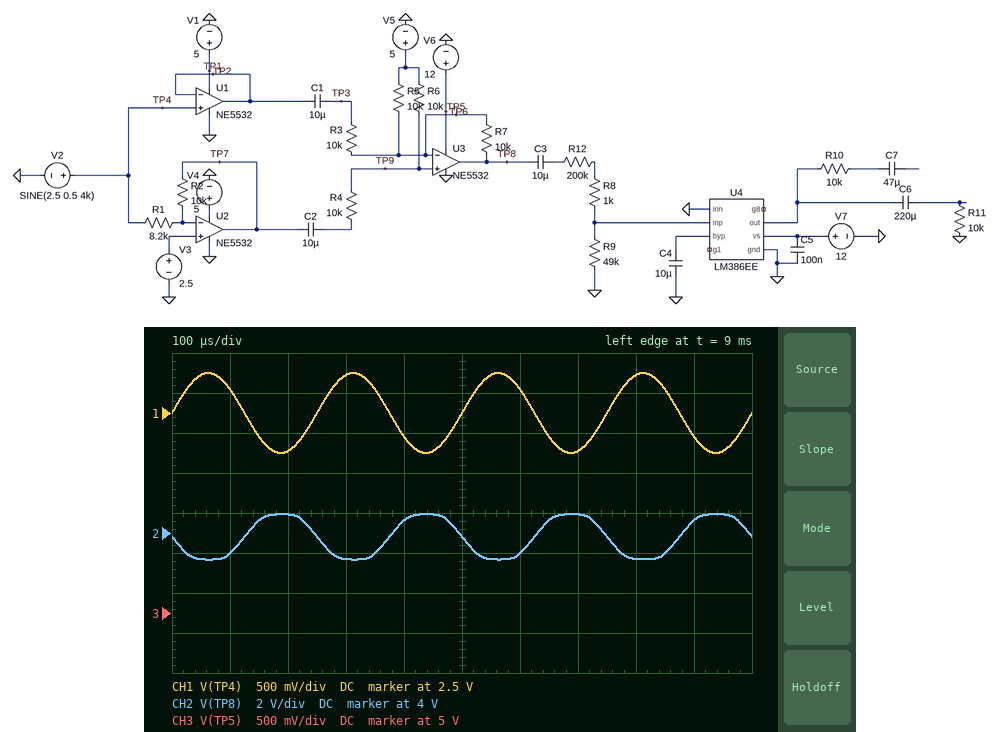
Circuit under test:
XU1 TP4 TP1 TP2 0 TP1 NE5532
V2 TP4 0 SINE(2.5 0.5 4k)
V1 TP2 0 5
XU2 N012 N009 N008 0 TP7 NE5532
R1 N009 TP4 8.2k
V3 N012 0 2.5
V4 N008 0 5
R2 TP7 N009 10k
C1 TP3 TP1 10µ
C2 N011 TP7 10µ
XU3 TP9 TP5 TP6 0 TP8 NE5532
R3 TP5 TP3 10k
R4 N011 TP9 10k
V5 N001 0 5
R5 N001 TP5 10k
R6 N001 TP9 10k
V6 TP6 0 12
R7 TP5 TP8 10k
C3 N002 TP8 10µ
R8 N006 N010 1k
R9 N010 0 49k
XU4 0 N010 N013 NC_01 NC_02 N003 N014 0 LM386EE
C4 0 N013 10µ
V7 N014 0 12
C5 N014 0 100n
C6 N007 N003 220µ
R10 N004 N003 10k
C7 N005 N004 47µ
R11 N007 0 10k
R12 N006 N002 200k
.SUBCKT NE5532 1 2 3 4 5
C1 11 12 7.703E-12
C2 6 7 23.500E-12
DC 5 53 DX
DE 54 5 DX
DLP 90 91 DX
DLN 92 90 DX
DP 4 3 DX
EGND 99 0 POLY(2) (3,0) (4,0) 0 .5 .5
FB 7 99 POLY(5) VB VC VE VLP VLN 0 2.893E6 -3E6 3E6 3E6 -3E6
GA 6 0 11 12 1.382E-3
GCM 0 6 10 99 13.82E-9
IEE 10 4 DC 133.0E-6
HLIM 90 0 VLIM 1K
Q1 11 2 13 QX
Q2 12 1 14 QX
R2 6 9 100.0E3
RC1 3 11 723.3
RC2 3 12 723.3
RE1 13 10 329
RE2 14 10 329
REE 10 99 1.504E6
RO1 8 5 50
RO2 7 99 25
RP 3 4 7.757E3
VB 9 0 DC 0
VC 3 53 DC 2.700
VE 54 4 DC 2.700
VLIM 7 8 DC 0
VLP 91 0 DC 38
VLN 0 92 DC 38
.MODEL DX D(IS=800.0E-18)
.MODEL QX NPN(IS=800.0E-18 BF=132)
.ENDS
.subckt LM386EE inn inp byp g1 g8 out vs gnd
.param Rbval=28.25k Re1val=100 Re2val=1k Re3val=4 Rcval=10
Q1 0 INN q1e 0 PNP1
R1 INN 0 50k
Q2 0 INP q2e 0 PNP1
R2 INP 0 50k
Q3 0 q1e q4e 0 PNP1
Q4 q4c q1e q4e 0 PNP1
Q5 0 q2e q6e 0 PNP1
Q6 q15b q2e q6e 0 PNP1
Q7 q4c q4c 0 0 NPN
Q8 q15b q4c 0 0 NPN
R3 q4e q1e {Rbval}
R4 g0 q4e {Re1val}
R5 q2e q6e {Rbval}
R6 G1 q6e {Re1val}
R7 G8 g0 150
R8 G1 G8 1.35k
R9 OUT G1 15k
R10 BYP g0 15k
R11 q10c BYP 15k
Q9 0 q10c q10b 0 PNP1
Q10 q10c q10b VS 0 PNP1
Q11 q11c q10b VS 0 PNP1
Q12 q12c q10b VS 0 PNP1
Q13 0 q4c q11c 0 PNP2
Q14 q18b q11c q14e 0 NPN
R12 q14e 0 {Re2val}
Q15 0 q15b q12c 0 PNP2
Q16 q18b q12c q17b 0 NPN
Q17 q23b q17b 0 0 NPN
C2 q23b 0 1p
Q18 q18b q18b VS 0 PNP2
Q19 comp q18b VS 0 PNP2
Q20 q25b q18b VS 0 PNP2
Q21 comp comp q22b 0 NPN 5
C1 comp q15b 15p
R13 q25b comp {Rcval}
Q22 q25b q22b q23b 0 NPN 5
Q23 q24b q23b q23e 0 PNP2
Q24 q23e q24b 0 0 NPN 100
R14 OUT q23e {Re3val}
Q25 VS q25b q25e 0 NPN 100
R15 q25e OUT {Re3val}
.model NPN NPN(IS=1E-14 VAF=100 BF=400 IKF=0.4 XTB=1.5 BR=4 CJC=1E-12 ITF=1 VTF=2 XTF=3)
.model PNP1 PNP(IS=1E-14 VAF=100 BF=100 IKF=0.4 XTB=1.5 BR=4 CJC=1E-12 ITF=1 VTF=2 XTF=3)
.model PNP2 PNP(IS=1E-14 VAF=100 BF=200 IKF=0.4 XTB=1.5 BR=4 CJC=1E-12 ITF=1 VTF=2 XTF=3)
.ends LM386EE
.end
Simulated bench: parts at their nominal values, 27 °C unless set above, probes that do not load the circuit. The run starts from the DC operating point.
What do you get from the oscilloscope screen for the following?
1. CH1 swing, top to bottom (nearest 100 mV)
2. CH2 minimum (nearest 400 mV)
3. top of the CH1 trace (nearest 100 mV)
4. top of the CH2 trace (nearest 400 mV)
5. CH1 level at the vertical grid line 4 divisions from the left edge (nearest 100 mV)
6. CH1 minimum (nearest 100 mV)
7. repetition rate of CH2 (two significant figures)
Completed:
1.0 V
2.8 V
3.0 V
4.8 V
2.2 V
2.0 V
4.0 kHz
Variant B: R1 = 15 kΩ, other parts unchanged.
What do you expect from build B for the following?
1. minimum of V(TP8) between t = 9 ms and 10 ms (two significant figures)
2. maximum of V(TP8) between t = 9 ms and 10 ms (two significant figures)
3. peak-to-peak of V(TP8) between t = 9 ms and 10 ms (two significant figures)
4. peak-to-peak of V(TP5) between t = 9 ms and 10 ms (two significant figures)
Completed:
2.9 V
4.8 V
1.9 V
340 mV
